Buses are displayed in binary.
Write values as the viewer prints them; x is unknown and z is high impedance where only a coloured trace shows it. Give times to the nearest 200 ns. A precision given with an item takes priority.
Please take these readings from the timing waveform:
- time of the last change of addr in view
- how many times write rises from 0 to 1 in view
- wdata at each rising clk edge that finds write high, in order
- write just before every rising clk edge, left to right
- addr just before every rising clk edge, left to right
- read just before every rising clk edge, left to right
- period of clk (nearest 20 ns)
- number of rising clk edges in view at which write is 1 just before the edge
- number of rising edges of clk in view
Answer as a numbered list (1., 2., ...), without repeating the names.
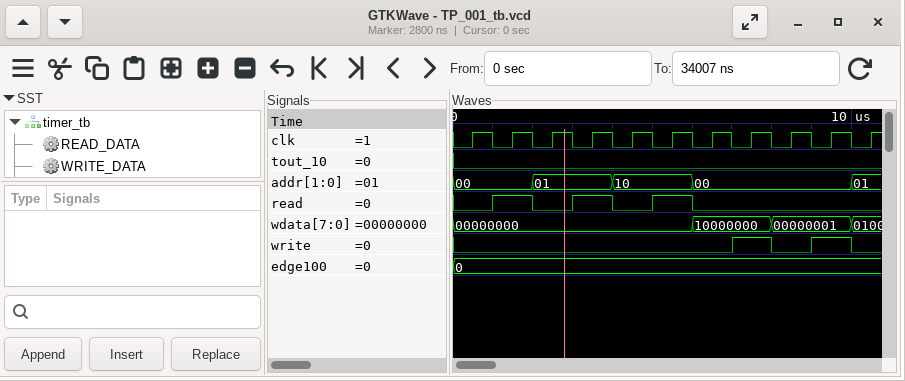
1. 10000 ns
2. 2
3. 10000000, 00000001
4. 0 0 0 0 0 0 0 1 0 1 0
5. 00, 00, 01, 01, 10, 10, 00, 00, 00, 00, 01
6. 0 1 0 1 0 1 0 0 0 0 0
7. 1000 ns
8. 2
9. 11
